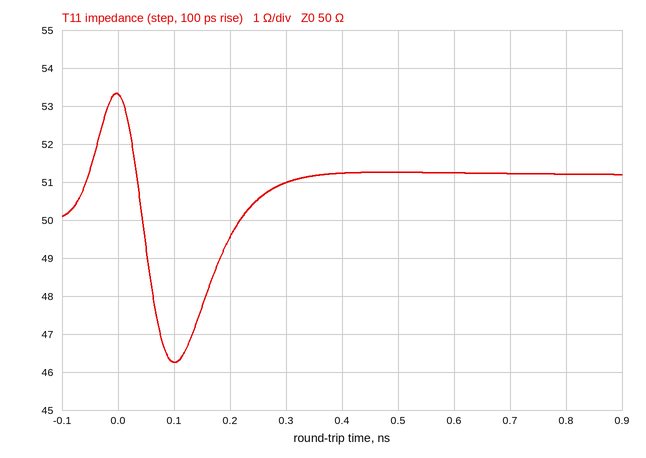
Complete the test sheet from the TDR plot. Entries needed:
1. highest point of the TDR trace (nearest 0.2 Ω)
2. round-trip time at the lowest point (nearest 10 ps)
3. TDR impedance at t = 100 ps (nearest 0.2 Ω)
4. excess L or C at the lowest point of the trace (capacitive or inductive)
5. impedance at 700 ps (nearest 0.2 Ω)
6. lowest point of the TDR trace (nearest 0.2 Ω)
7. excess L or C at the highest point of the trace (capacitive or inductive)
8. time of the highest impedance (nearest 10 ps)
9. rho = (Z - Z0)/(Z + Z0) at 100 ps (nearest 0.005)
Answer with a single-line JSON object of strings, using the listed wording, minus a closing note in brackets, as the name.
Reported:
{"highest point of the TDR trace": "53.4 Ω", "round-trip time at the lowest point": "100 ps", "TDR impedance at t = 100 ps": "46.2 Ω", "excess L or C at the lowest point of the trace": "capacitive", "impedance at 700 ps": "51.2 Ω", "lowest point of the TDR trace": "46.2 Ω", "excess L or C at the highest point of the trace": "inductive", "time of the highest impedance": "0 ps", "rho = (Z - Z0)/(Z + Z0) at 100 ps": "-0.040"}
